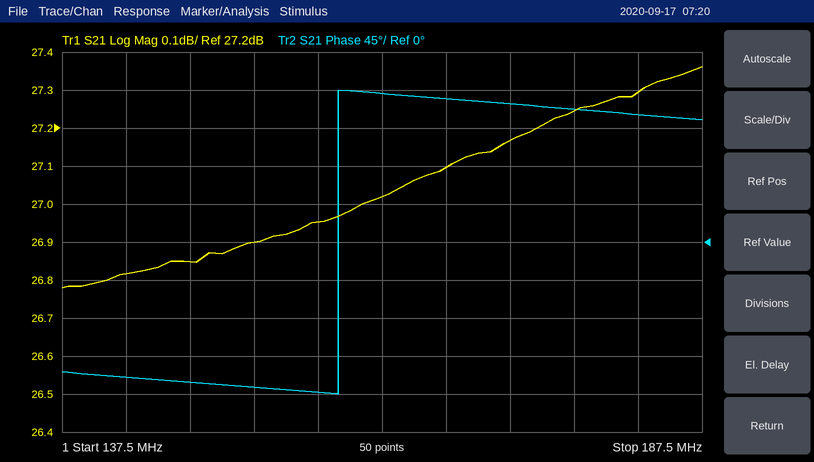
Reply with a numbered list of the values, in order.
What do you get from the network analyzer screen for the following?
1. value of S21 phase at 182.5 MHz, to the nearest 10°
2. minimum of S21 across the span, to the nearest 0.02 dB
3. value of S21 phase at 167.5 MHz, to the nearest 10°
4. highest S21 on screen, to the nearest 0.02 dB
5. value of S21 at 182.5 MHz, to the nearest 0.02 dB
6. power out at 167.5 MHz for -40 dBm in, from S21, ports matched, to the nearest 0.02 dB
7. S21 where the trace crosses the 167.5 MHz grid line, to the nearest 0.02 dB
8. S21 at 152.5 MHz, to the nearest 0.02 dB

1. 150°
2. 26.78 dB
3. 170°
4. 27.36 dB
5. 27.30 dB
6. -12.90 dBm
7. 27.10 dB
8. 26.90 dB
